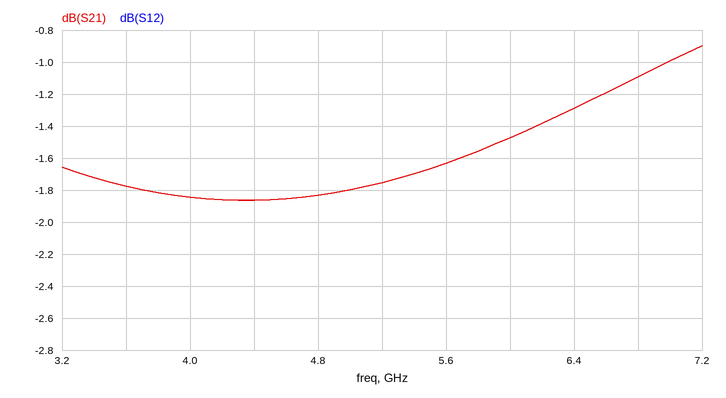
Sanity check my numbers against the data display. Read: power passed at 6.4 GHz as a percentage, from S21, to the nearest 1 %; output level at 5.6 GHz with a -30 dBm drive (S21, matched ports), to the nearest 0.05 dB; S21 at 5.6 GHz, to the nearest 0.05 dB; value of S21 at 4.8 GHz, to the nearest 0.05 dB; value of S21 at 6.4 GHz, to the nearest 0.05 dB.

74 %
-31.65 dBm
-1.65 dB
-1.85 dB
-1.30 dB
